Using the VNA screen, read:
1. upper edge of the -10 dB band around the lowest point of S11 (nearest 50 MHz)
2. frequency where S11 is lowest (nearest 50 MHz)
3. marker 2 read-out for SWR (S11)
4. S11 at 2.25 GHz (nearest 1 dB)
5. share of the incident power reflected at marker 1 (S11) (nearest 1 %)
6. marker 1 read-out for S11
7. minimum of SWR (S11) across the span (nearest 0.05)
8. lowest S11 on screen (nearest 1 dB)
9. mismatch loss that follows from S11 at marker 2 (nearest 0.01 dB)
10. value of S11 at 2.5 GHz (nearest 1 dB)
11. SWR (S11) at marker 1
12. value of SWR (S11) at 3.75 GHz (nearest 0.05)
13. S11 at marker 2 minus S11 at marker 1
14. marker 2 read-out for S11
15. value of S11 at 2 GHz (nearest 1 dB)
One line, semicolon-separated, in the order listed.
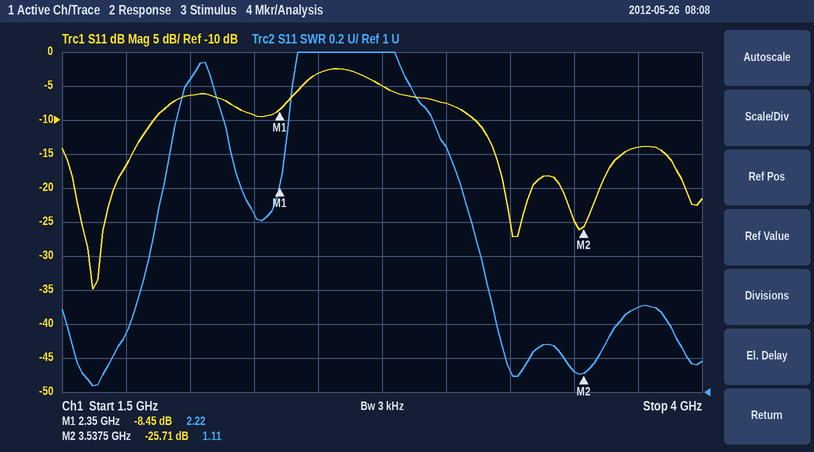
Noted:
1.85 GHz; 1.60 GHz; 1.11; -9 dB; 14 %; -8.45 dB; 1.05; -35 dB; 0.01 dB; -3 dB; 2.22; 1.50; -17.26 dB; -25.71 dB; -6 dB
